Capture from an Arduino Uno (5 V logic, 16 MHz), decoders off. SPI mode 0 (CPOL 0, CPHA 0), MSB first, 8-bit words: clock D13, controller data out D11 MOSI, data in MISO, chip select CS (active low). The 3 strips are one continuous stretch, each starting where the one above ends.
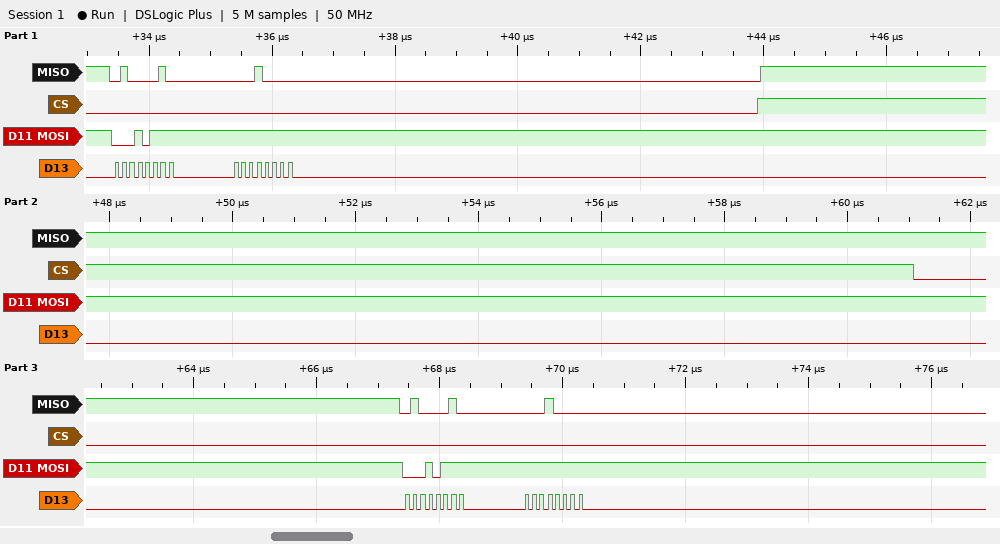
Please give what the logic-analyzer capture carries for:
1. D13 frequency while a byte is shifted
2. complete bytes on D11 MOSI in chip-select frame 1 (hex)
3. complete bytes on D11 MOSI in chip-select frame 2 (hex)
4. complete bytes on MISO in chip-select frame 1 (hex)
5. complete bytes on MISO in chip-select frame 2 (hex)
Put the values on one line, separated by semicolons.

8 MHz; 17 FF; 17 FF; 42 10; 42 10
